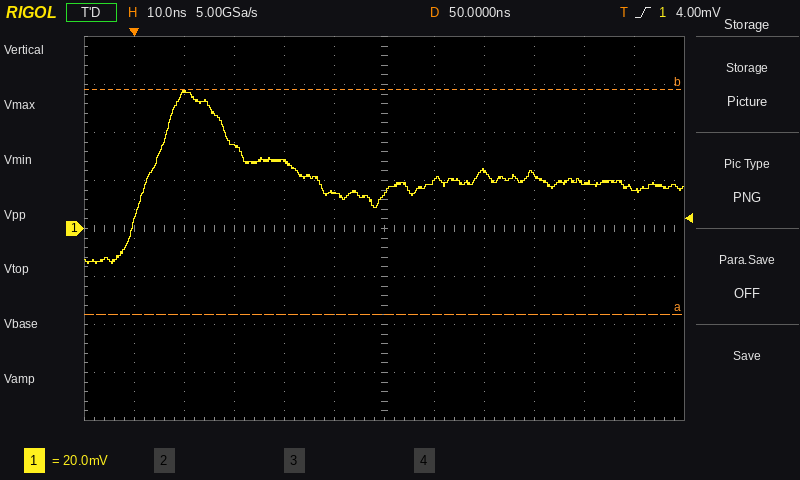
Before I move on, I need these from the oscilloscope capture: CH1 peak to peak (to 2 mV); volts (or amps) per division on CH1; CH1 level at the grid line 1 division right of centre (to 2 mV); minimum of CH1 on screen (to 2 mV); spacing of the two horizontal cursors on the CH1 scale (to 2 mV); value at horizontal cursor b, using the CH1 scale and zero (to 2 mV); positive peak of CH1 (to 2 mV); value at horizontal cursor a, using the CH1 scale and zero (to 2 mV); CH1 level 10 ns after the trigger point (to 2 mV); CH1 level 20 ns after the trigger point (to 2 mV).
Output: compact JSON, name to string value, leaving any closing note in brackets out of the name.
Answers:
{"CH1 peak to peak": "72 mV", "volts (or amps) per division on CH1": "20 mV", "CH1 level at the grid line 1 division right of centre": "20 mV", "minimum of CH1 on screen": "-14 mV", "spacing of the two horizontal cursors on the CH1 scale": "94 mV", "value at horizontal cursor b, using the CH1 scale and zero": "58 mV", "positive peak of CH1": "58 mV", "value at horizontal cursor a, using the CH1 scale and zero": "-36 mV", "CH1 level 10 ns after the trigger point": "56 mV", "CH1 level 20 ns after the trigger point": "34 mV"}
